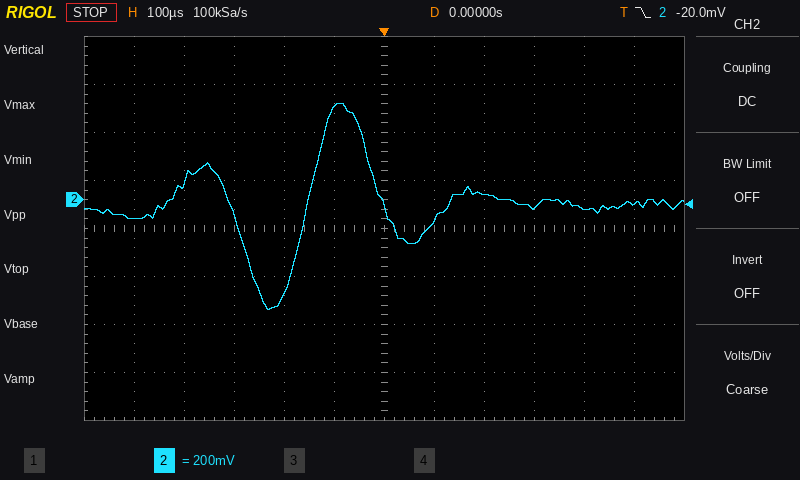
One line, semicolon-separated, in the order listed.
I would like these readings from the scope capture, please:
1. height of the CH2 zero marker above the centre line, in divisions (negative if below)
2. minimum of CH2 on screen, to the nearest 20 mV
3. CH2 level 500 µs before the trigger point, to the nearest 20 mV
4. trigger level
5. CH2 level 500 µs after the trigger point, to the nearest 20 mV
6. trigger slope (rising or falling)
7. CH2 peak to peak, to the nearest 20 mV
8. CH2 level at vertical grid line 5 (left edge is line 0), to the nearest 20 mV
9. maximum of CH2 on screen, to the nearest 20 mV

+0.6 div; -460 mV; -80 mV; -20.0 mV; -20 mV; falling; 860 mV; 380 mV; 400 mV
